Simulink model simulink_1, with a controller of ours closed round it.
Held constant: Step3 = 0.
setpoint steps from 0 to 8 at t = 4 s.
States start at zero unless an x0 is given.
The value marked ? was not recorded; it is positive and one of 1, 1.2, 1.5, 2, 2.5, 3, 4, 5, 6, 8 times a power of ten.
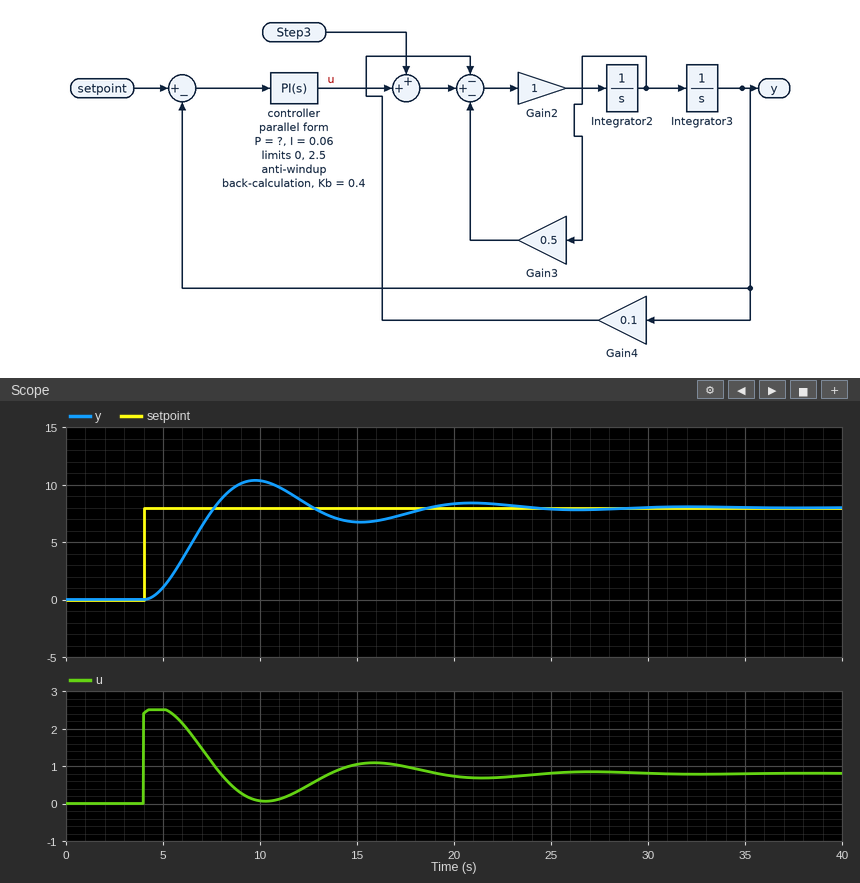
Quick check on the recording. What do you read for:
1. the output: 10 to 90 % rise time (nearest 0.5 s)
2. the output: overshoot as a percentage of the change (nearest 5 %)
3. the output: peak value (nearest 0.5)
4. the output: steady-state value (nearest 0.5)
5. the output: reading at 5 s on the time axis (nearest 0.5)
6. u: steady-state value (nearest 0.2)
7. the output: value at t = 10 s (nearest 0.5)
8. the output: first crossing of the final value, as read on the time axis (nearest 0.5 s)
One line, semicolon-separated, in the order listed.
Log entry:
2.5 s; 30 %; 10.5; 8.0; 1.0; 0.8; 10.5; 7.5 s
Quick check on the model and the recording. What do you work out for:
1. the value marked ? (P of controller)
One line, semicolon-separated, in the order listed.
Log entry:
0.3
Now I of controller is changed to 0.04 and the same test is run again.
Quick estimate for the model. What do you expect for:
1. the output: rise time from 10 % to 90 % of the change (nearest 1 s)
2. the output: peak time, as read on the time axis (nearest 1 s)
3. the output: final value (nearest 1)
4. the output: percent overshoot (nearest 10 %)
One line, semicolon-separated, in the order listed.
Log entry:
3 s; 10 s; 8; 20 %
